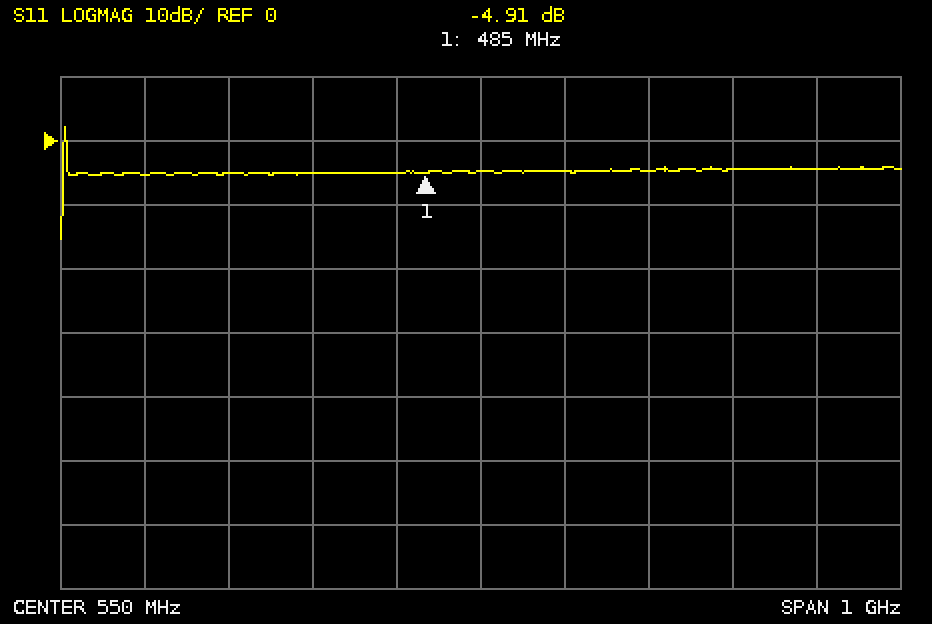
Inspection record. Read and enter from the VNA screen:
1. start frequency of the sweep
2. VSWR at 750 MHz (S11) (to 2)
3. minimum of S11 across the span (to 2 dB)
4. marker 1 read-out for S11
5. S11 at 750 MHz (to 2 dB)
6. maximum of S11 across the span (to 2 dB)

50 MHz
4
-16 dB
-4.91 dB
-4 dB
2 dB
